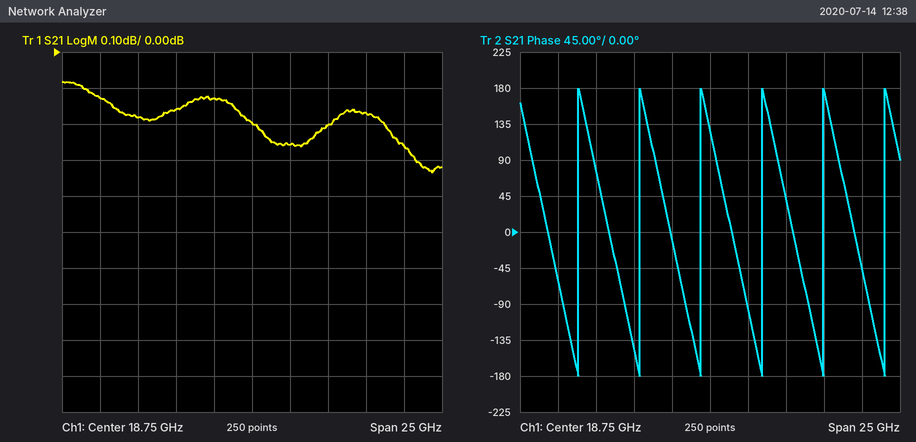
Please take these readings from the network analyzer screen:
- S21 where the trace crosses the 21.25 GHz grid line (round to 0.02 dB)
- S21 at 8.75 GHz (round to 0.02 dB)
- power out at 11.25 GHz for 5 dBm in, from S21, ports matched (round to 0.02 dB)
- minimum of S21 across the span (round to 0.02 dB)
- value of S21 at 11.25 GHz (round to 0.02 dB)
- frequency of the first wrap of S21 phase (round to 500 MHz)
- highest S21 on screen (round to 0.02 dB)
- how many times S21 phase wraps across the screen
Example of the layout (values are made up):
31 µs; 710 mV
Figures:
-0.26 dB; -0.12 dB; 4.82 dBm; -0.34 dB; -0.18 dB; 10.0 GHz; -0.08 dB; 6
